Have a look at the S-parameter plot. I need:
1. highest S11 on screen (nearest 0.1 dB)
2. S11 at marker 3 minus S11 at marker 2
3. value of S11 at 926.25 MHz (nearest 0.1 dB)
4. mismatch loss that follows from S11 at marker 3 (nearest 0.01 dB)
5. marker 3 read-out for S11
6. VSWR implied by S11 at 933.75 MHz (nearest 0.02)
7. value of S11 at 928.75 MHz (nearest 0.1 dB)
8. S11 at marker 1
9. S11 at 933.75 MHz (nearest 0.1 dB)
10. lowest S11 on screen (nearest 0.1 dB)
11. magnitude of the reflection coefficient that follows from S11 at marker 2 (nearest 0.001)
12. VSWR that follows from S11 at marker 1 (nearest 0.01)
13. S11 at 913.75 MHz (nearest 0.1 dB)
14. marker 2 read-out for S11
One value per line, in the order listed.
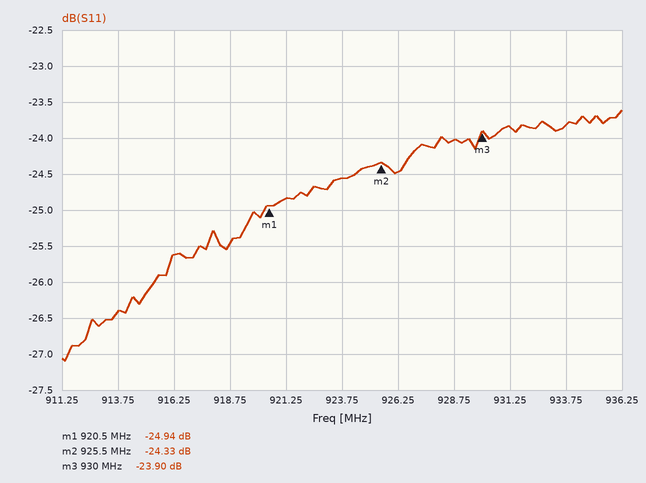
-23.6 dB
0.43 dB
-24.5 dB
0.02 dB
-23.90 dB
1.14
-24.0 dB
-24.94 dB
-23.8 dB
-27.1 dB
0.061
1.12
-26.4 dB
-24.33 dB
